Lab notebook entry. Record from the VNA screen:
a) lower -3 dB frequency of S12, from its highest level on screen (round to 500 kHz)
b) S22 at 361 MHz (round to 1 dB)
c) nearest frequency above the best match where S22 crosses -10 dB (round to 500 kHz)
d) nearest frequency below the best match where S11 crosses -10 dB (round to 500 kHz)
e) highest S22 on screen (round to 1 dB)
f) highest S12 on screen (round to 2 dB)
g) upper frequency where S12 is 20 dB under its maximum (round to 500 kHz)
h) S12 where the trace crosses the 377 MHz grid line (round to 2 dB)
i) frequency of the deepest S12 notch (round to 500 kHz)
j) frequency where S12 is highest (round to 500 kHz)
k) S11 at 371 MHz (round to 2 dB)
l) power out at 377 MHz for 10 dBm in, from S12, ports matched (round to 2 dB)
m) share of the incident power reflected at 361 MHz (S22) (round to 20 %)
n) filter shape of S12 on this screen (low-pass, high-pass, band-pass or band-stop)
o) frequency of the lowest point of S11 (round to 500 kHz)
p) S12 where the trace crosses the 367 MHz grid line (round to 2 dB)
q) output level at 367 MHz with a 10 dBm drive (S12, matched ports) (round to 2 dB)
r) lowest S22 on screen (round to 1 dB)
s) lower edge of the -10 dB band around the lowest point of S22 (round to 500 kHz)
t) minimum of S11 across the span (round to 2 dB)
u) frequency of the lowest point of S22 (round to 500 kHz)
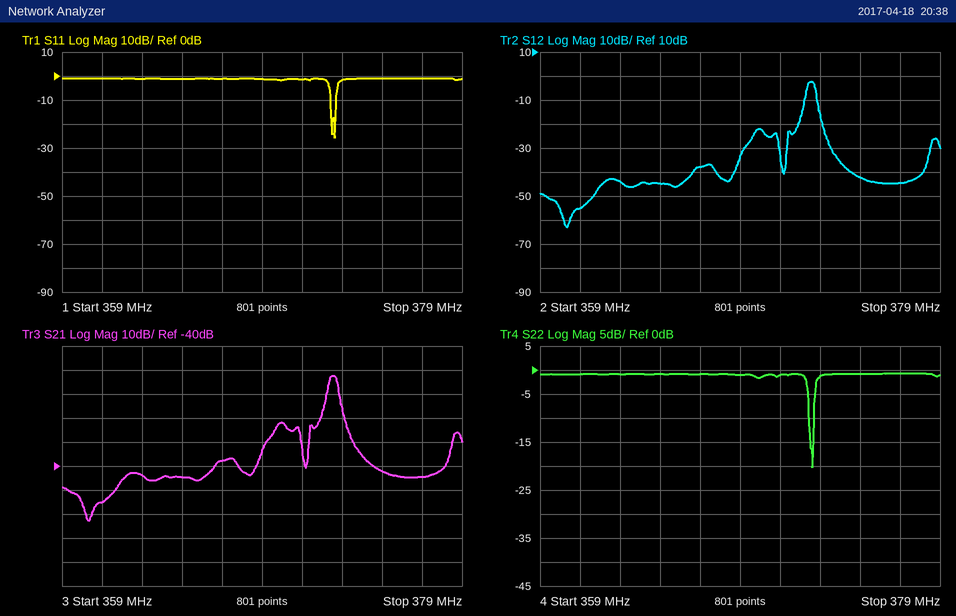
372.5 MHz
-1 dB
372.5 MHz
372.5 MHz
-1 dB
-2 dB
373.0 MHz
-44 dB
360.5 MHz
372.5 MHz
-2 dB
-34 dBm
80 %
band-pass
372.5 MHz
-38 dB
-28 dBm
-20 dB
372.5 MHz
-26 dB
372.5 MHz
